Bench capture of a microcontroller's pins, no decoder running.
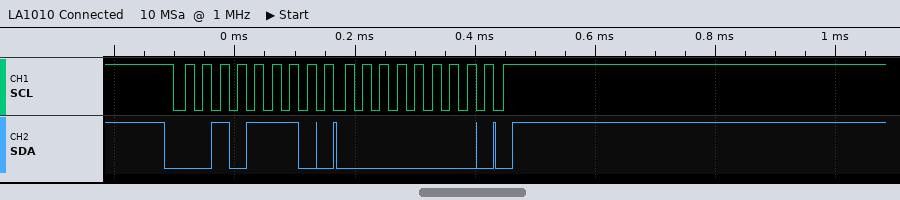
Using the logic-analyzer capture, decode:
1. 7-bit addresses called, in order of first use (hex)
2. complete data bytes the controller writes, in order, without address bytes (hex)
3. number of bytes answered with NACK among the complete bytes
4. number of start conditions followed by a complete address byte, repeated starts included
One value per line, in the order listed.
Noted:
0x17
00
0
1
